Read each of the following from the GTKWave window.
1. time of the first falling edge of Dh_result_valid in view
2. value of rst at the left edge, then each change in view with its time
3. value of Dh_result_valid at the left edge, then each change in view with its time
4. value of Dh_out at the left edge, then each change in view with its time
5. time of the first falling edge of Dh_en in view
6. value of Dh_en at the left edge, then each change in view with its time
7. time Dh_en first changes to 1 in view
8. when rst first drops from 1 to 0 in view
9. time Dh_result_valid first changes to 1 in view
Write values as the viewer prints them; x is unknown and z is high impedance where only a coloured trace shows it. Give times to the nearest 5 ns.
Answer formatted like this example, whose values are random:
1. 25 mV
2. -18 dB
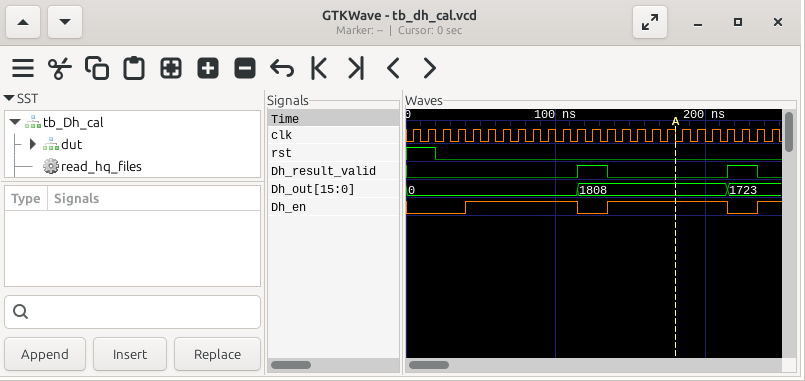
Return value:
1. 135 ns
2. 1, 0 at 20 ns
3. 0, 1 at 115 ns, 0 at 135 ns, 1 at 215 ns, 0 at 235 ns
4. 0, 1808 at 115 ns, 1723 at 215 ns
5. 115 ns
6. 0, 1 at 40 ns, 0 at 115 ns, 1 at 135 ns, 0 at 215 ns, 1 at 235 ns
7. 40 ns
8. 20 ns
9. 115 ns
